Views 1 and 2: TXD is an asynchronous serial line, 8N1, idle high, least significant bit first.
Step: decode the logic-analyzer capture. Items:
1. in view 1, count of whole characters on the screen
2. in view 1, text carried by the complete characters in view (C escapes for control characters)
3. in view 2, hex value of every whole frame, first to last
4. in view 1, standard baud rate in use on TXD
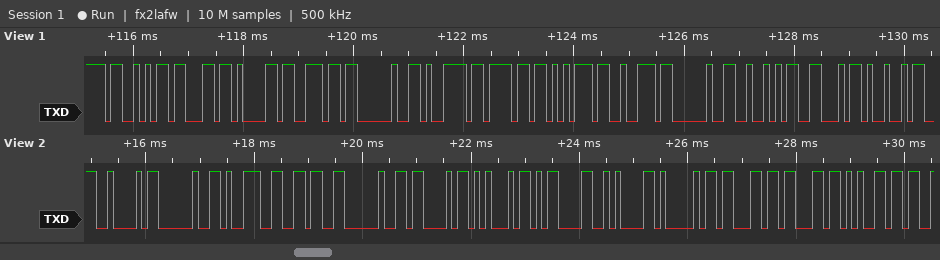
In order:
13
"Scan your RFI"
42 20 39 36 20 43 45 0D 0A 41 63 63 65
9600 baud
